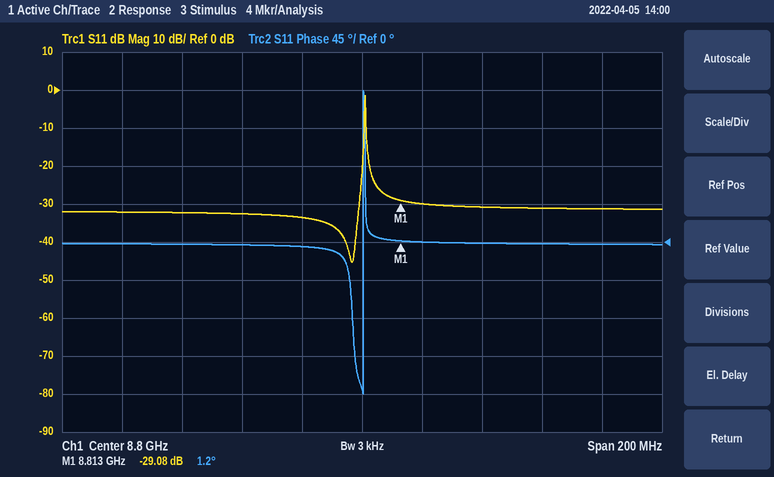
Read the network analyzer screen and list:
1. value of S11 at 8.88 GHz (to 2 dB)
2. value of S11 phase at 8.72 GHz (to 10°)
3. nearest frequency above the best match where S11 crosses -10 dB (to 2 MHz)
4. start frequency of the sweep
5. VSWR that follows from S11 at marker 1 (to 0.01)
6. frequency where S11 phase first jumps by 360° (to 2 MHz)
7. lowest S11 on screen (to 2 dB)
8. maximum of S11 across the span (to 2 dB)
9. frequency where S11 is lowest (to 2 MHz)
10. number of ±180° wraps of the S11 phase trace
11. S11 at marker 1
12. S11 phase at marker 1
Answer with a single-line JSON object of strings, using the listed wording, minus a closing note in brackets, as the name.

{"value of S11 at 8.88 GHz": "-32 dB", "value of S11 phase at 8.72 GHz": "0°", "nearest frequency above the best match where S11 crosses -10 dB": "8.800 GHz", "start frequency of the sweep": "8.7 GHz", "VSWR that follows from S11 at marker 1": "1.07", "frequency where S11 phase first jumps by 360°": "8.800 GHz", "lowest S11 on screen": "-46 dB", "maximum of S11 across the span": "-2 dB", "frequency where S11 is lowest": "8.796 GHz", "number of ±180° wraps of the S11 phase trace": "1", "S11 at marker 1": "-29.08 dB", "S11 phase at marker 1": "1.2°"}
